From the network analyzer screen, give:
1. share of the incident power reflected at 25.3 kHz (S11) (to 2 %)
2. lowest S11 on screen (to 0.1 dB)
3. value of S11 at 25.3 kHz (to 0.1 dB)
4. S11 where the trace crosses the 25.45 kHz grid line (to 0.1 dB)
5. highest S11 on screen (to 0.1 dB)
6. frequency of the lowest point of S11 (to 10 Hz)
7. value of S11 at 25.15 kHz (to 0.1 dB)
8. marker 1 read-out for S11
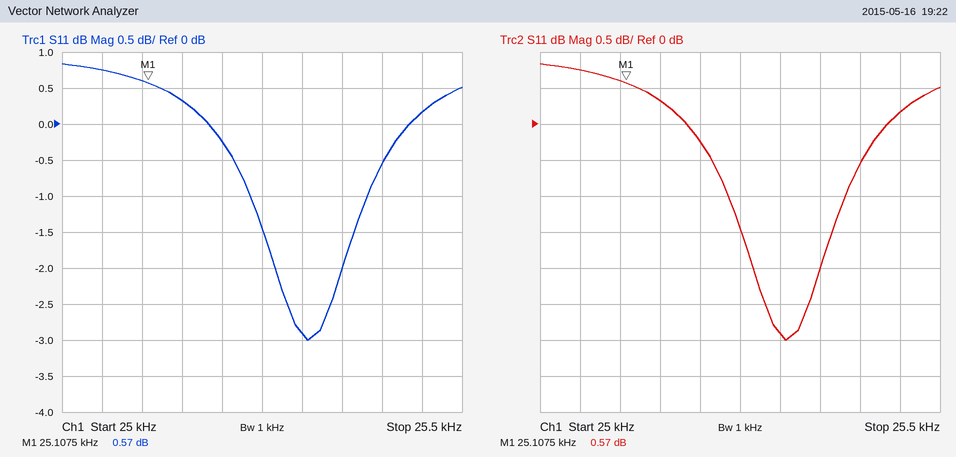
52 %
-3.0 dB
-2.9 dB
0.2 dB
0.8 dB
25.31 kHz
0.3 dB
0.57 dB
